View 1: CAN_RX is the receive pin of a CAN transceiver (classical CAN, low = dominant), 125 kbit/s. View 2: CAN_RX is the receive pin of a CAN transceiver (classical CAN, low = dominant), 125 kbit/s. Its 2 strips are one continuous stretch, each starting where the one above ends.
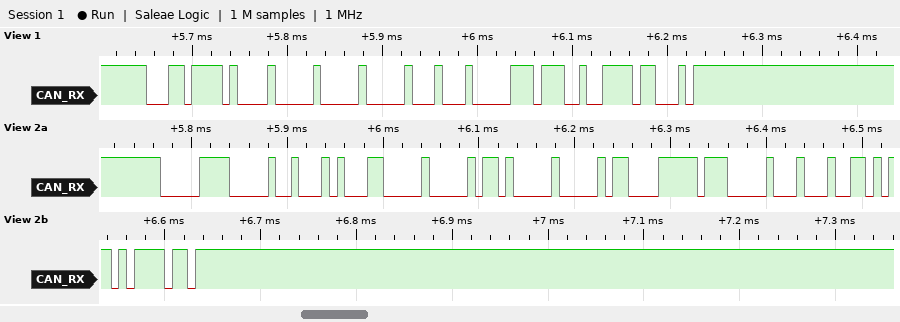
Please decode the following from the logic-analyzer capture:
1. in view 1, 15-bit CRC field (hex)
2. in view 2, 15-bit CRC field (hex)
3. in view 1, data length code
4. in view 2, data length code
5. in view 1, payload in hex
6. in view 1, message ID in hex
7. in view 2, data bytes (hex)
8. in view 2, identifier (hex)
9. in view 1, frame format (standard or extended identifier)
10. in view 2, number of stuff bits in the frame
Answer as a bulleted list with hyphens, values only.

- 0x13D8
- 0x56BD
- 4
- 8
- 00 00 88 37
- 0x1BD
- A3 00 1A 00 30 FF 00 89
- 0x070
- standard
- 8
